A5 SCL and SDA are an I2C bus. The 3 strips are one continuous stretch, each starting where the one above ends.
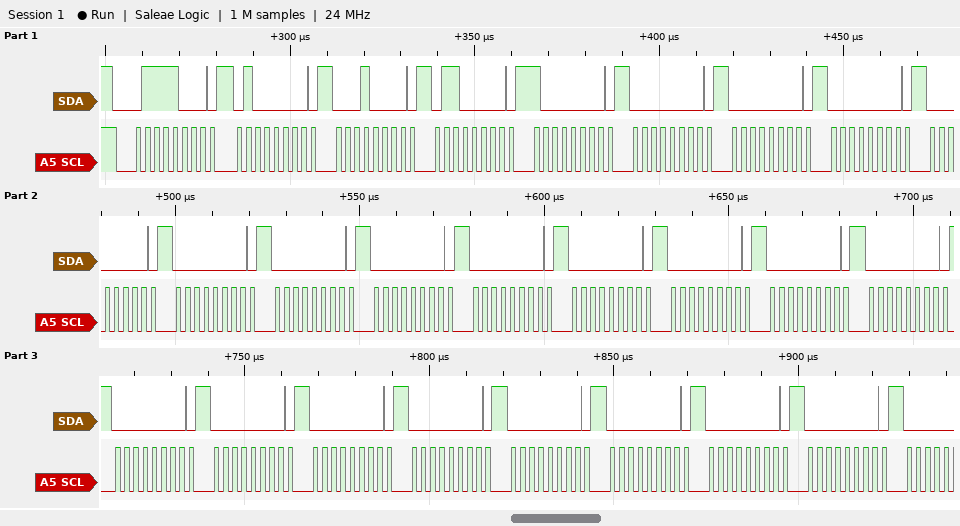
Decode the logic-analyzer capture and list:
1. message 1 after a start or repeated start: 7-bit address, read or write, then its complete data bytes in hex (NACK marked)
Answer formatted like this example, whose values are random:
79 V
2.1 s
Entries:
0x3C write: 40 10 60 80 00 00 00 00 00 00 00 00 00 00 00 00 00 00 00 00 00 00 00 00
